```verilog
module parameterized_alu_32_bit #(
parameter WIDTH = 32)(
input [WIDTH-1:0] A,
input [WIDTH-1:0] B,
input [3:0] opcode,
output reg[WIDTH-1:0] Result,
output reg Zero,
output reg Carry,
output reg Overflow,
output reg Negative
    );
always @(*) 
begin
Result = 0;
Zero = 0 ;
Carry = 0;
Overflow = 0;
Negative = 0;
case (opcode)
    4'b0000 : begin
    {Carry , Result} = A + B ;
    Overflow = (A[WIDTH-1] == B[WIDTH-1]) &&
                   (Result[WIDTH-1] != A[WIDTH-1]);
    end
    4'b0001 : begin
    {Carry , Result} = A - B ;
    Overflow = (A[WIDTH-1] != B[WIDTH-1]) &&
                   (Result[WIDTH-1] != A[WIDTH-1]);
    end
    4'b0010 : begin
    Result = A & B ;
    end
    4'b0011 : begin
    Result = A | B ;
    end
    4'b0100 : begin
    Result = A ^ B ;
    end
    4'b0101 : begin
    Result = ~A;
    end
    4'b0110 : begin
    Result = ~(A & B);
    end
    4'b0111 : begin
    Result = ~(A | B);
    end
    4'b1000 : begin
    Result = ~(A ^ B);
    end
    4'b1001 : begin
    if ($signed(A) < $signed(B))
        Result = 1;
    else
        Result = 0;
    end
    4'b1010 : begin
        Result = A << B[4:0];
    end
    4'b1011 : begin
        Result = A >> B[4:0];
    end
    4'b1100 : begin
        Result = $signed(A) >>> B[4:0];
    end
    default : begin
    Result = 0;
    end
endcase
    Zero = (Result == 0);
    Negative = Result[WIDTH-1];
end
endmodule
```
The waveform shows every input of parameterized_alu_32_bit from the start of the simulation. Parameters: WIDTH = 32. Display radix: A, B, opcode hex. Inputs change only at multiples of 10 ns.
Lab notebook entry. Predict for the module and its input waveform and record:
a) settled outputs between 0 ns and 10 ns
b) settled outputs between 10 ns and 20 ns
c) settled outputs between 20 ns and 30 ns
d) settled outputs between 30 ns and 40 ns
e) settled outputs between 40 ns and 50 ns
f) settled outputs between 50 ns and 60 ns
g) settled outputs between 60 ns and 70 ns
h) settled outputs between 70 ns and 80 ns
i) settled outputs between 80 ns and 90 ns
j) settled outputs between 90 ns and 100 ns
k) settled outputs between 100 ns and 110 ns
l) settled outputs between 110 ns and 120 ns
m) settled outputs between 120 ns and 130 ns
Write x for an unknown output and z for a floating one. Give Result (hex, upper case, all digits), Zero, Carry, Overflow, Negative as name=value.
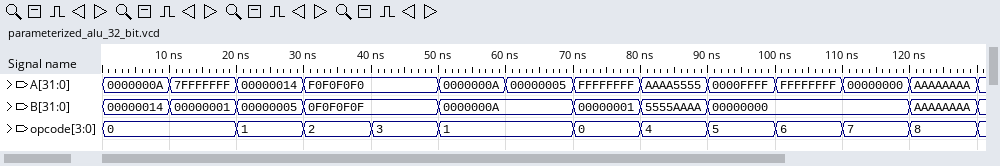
Result=0000001E, Zero=0, Carry=0, Overflow=0, Negative=0
Result=80000000, Zero=0, Carry=0, Overflow=1, Negative=1
Result=0000000F, Zero=0, Carry=0, Overflow=0, Negative=0
Result=00000000, Zero=1, Carry=0, Overflow=0, Negative=0
Result=FFFFFFFF, Zero=0, Carry=0, Overflow=0, Negative=1
Result=00000000, Zero=1, Carry=0, Overflow=0, Negative=0
Result=FFFFFFFB, Zero=0, Carry=1, Overflow=0, Negative=1
Result=00000000, Zero=1, Carry=1, Overflow=0, Negative=0
Result=FFFFFFFF, Zero=0, Carry=0, Overflow=0, Negative=1
Result=FFFF0000, Zero=0, Carry=0, Overflow=0, Negative=1
Result=FFFFFFFF, Zero=0, Carry=0, Overflow=0, Negative=1
Result=FFFFFFFF, Zero=0, Carry=0, Overflow=0, Negative=1
Result=FFFFFFFF, Zero=0, Carry=0, Overflow=0, Negative=1
